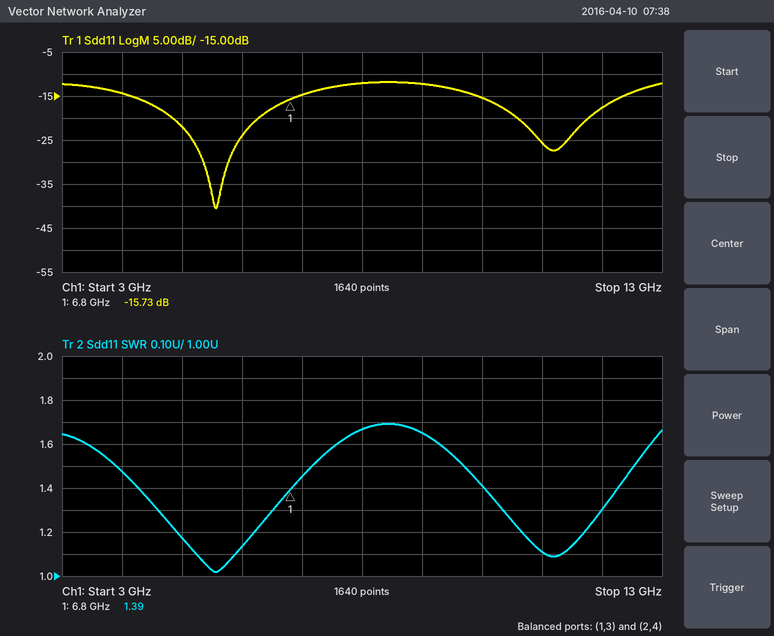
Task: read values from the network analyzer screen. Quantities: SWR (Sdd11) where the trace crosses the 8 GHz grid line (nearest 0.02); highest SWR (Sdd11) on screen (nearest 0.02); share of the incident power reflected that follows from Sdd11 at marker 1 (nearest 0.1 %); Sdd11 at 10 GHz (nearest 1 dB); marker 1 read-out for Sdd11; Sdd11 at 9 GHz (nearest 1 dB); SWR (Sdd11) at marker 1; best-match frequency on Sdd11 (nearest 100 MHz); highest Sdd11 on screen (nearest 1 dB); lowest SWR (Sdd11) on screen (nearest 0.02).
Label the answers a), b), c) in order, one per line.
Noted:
a) 1.66
b) 1.70
c) 2.7 %
d) -15 dB
e) -15.73 dB
f) -12 dB
g) 1.39
h) 5.6 GHz
i) -12 dB
j) 1.02
